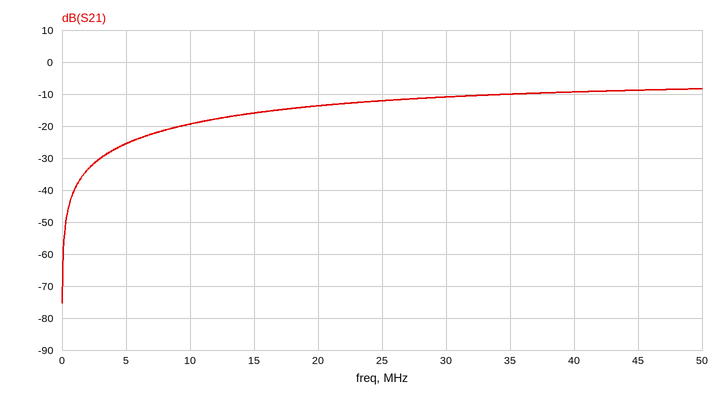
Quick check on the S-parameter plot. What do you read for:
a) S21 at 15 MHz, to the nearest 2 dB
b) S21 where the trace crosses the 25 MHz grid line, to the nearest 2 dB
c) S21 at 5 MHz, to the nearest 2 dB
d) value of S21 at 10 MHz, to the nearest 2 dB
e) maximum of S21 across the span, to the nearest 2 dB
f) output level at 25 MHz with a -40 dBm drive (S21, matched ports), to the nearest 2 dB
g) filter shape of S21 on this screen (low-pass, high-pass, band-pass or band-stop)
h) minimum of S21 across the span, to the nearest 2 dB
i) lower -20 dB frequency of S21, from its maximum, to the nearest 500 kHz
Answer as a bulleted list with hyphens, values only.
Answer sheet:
- -16 dB
- -12 dB
- -26 dB
- -20 dB
- -8 dB
- -52 dBm
- high-pass
- -76 dB
- 3.5 MHz
